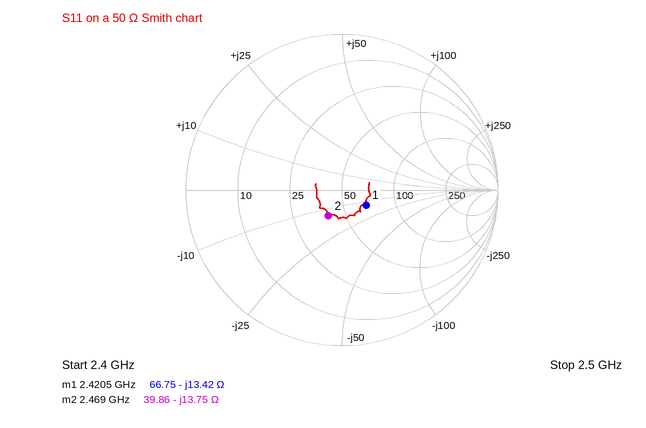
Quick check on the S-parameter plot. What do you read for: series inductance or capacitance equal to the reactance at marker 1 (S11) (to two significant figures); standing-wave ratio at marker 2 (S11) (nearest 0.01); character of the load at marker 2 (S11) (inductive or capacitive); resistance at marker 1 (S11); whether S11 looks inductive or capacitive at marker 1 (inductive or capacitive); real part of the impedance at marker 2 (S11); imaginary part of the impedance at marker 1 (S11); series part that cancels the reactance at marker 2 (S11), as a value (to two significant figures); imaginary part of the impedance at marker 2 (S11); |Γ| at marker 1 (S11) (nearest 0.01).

4.9 pF
1.46
capacitive
66.75 Ω
capacitive
39.86 Ω
-13.42 Ω
890 pH
-13.75 Ω
0.18
